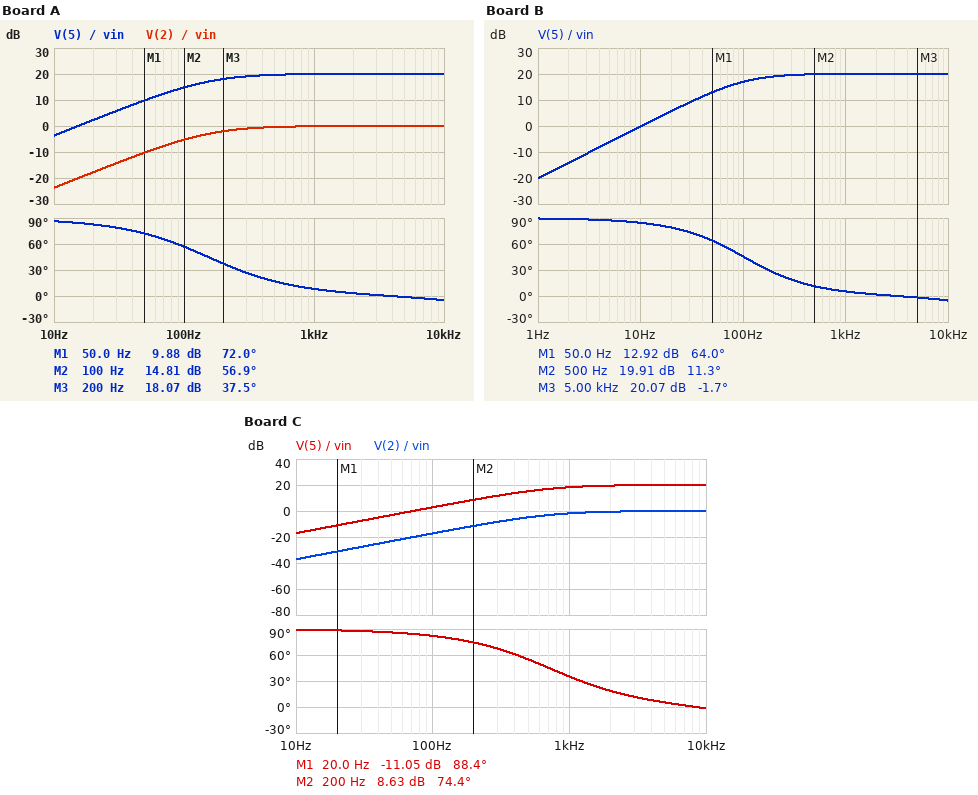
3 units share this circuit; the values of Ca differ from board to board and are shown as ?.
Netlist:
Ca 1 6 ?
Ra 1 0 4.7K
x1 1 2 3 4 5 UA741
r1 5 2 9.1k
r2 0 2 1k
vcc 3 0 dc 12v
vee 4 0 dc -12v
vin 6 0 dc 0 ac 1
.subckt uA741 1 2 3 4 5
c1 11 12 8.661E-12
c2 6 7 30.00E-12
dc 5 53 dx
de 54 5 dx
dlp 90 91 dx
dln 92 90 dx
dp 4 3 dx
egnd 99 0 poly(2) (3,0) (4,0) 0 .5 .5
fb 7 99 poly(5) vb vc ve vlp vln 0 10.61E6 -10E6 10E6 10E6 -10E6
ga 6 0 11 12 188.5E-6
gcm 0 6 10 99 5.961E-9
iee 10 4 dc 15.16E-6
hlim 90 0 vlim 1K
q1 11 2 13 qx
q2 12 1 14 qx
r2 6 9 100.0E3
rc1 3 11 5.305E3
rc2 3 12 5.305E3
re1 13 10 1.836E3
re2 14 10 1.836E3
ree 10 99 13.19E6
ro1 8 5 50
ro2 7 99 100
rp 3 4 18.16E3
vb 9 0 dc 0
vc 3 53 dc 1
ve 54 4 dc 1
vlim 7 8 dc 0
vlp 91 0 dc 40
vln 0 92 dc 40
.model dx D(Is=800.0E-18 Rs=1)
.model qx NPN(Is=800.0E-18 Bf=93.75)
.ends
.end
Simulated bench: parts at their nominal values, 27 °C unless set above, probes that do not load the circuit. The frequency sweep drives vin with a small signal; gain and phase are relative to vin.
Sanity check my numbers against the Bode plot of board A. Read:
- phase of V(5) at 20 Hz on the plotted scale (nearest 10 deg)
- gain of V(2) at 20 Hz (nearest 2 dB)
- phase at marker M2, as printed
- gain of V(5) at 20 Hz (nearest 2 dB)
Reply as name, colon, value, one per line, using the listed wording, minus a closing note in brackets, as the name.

phase of V(5) at 20 Hz on the plotted scale: 80 deg
gain of V(2) at 20 Hz: -18 dB
phase at marker M2, as printed: 56.9 deg
gain of V(5) at 20 Hz: 2 dB
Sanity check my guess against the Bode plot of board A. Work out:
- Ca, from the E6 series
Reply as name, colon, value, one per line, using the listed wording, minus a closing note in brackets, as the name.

Ca, from the E6 series: 220 nF
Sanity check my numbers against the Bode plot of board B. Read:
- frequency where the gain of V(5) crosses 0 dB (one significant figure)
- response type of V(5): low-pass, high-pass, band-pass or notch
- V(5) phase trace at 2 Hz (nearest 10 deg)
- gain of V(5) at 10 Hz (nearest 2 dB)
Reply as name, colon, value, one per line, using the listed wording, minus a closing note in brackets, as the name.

frequency where the gain of V(5) crosses 0 dB: 10 Hz
response type of V(5): low-pass, high-pass, band-pass or notch: high-pass
V(5) phase trace at 2 Hz: 90 deg
gain of V(5) at 10 Hz: 0 dB
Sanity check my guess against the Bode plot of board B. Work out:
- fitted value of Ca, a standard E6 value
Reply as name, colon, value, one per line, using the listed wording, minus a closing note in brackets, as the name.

fitted value of Ca, a standard E6 value: 330 nF
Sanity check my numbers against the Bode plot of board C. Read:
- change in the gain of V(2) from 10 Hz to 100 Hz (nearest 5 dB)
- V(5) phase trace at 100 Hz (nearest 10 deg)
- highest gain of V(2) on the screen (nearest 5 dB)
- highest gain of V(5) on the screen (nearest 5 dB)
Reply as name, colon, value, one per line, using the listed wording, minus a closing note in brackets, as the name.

change in the gain of V(2) from 10 Hz to 100 Hz: 20 dB
V(5) phase trace at 100 Hz: 80 deg
highest gain of V(2) on the screen: 0 dB
highest gain of V(5) on the screen: 20 dB
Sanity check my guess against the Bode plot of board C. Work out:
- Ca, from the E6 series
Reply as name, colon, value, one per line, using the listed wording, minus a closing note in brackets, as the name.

Ca, from the E6 series: 47 nF
